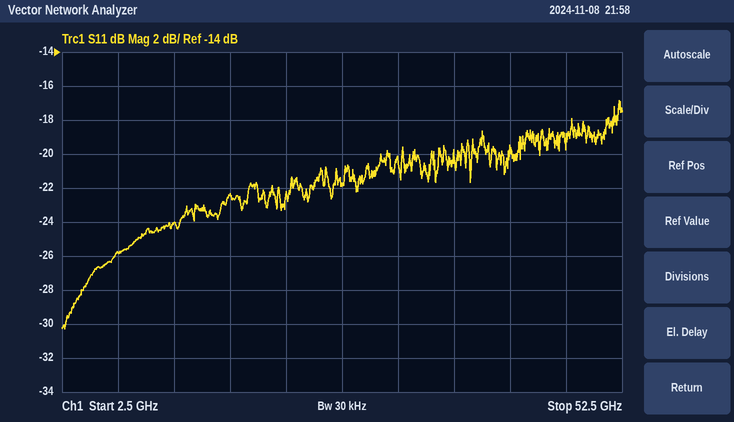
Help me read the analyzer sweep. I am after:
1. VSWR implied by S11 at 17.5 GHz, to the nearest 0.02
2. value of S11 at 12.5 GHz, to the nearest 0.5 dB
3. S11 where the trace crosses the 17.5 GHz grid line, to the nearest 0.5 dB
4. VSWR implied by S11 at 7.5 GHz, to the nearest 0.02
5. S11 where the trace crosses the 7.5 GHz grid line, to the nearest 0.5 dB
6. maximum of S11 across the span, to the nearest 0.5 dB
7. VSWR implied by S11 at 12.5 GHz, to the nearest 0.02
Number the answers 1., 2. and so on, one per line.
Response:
1. 1.16
2. -24.0 dB
3. -22.5 dB
4. 1.10
5. -26.0 dB
6. -17.0 dB
7. 1.14
